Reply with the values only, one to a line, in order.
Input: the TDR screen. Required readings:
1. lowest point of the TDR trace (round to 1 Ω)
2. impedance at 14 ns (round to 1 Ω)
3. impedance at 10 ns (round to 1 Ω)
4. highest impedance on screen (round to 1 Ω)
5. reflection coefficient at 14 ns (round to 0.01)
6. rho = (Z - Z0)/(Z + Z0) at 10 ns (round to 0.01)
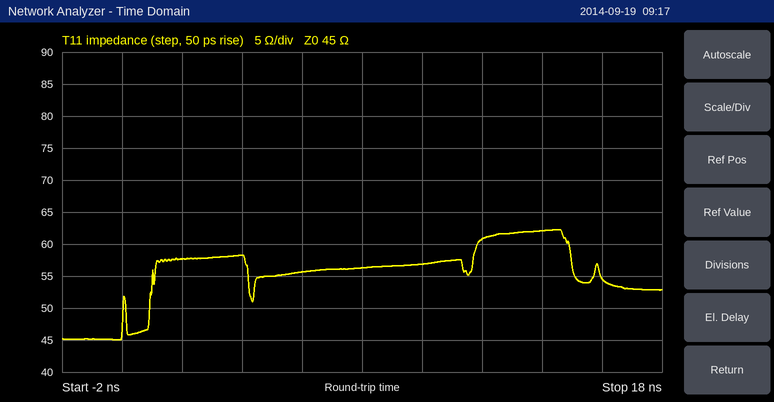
45 Ω
62 Ω
57 Ω
62 Ω
+0.16
+0.12
